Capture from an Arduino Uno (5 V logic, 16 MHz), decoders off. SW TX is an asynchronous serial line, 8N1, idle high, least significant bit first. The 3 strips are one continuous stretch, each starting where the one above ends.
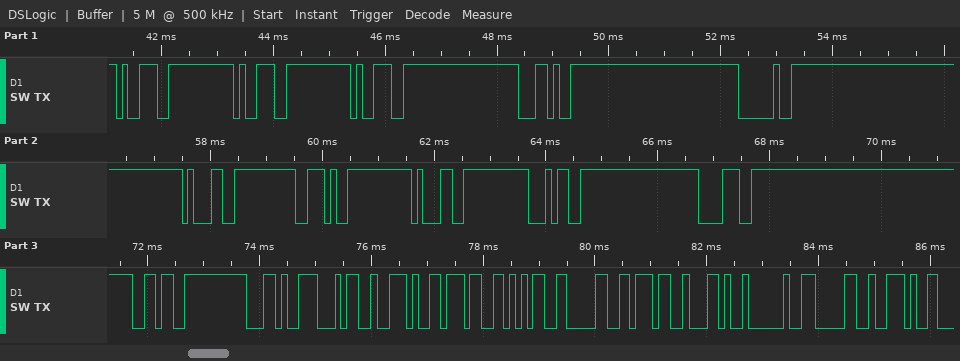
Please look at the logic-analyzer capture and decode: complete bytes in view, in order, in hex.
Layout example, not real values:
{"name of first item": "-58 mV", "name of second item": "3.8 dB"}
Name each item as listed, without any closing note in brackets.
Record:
{"complete bytes in view, in order, in hex": "39 39 39 2C 20 31 2E 31 34 38 36 2C 34 2E 37 35 30 37 2C 20 30 2E"}
